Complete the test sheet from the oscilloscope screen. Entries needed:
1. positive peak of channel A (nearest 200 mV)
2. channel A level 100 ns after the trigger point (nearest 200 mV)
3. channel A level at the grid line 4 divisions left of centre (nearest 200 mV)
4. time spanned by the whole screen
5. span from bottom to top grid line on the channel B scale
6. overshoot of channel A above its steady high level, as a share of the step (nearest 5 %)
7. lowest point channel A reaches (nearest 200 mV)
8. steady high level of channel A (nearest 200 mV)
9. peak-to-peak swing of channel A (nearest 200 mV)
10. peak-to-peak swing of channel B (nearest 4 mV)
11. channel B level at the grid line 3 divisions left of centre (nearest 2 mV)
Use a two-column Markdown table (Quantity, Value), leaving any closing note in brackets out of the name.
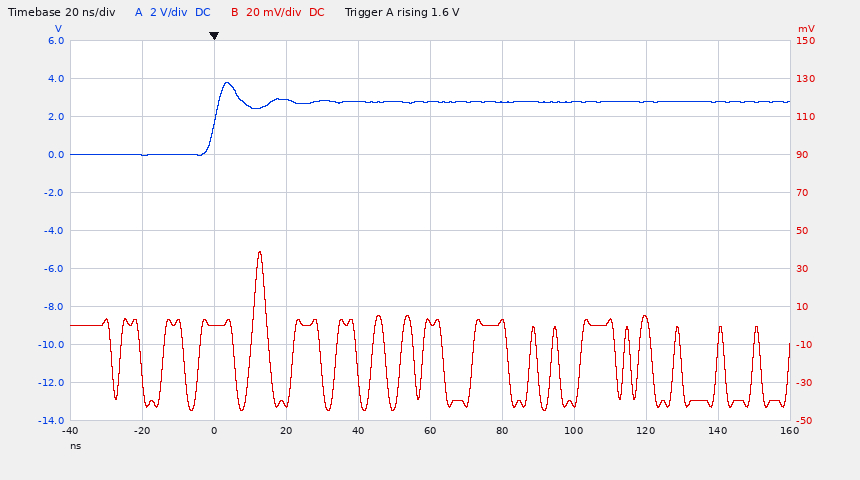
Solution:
| Quantity | Value |
|---|---|
| positive peak of channel A | 3.8 V |
| channel A level 100 ns after the trigger point | 2.8 V |
| channel A level at the grid line 4 divisions left of centre | 0.0 V |
| time spanned by the whole screen | 200 ns |
| span from bottom to top grid line on the channel B scale | 200 mV |
| overshoot of channel A above its steady high level, as a share of the step | 35 % |
| lowest point channel A reaches | 0.0 V |
| steady high level of channel A | 2.8 V |
| peak-to-peak swing of channel A | 3.8 V |
| peak-to-peak swing of channel B | 84 mV |
| channel B level at the grid line 3 divisions left of centre | 0 mV |
